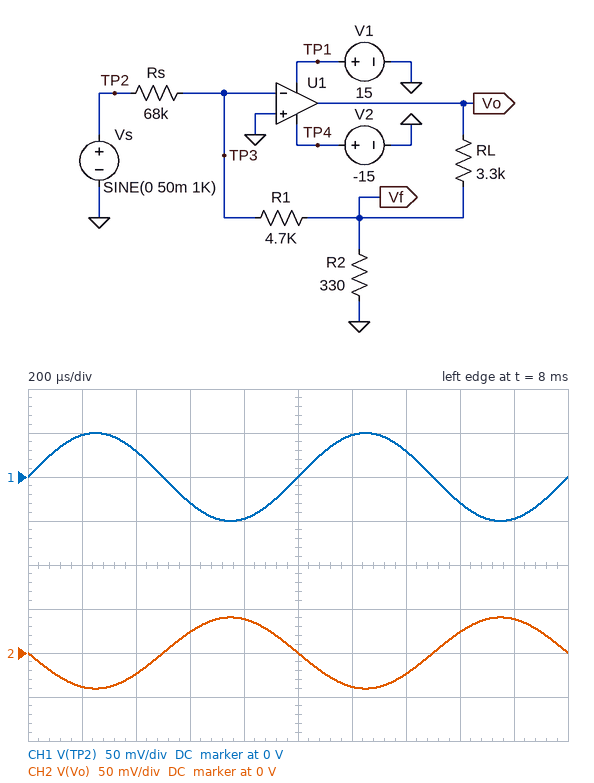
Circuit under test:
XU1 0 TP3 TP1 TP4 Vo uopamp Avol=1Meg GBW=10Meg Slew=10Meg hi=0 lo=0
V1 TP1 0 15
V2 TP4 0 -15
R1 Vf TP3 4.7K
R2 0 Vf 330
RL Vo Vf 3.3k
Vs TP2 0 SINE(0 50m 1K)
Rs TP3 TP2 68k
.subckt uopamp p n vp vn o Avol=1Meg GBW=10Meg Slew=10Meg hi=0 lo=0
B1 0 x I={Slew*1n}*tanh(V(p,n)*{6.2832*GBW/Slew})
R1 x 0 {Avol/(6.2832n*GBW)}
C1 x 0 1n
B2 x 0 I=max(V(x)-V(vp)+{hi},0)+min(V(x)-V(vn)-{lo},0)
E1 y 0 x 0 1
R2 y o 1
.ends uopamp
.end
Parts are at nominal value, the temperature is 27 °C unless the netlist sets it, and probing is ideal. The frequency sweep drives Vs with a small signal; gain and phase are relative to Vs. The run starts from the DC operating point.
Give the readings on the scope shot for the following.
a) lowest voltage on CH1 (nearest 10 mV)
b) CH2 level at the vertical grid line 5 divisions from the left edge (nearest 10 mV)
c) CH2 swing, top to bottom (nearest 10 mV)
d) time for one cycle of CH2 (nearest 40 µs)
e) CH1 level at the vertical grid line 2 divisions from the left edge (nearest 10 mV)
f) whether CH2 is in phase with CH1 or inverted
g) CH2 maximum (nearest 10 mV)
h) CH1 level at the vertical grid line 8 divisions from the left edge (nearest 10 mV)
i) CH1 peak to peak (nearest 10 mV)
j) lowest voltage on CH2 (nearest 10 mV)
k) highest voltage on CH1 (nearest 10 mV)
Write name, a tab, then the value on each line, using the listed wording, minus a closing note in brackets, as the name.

lowest voltage on CH1	-50 mV
CH2 level at the vertical grid line 5 divisions from the left edge	0 V
CH2 swing, top to bottom	80 mV
time for one cycle of CH2	1.00 ms
CH1 level at the vertical grid line 2 divisions from the left edge	30 mV
whether CH2 is in phase with CH1 or inverted	inverted
CH2 maximum	40 mV
CH1 level at the vertical grid line 8 divisions from the left edge	-30 mV
CH1 peak to peak	100 mV
lowest voltage on CH2	-40 mV
highest voltage on CH1	50 mV
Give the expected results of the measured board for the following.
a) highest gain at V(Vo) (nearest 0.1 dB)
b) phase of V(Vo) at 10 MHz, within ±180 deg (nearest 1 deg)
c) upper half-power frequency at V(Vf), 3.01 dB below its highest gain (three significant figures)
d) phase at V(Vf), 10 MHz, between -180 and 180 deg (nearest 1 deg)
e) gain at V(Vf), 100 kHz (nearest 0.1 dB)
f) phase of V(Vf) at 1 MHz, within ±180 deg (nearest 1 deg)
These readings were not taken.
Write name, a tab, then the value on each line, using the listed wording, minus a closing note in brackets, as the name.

highest gain at V(Vo)	-1.8 dB
phase of V(Vo) at 10 MHz, within ±180 deg	95 deg
upper half-power frequency at V(Vf), 3.01 dB below its highest gain	850 kHz
phase at V(Vf), 10 MHz, between -180 and 180 deg	60 deg
gain at V(Vf), 100 kHz	-23.3 dB
phase of V(Vf) at 1 MHz, within ±180 deg	126 deg
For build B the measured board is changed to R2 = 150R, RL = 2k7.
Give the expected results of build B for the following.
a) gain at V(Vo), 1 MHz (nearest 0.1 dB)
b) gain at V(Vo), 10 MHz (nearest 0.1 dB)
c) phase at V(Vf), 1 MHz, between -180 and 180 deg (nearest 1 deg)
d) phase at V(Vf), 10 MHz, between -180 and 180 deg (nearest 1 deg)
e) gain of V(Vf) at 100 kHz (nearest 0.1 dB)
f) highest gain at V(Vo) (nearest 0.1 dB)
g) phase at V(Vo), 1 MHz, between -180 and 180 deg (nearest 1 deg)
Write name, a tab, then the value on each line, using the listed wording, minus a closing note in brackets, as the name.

gain at V(Vo), 1 MHz	-4.5 dB
gain at V(Vo), 10 MHz	-23.6 dB
phase at V(Vf), 1 MHz, between -180 and 180 deg	113 deg
phase at V(Vf), 10 MHz, between -180 and 180 deg	63 deg
gain of V(Vf) at 100 kHz	-23.4 dB
highest gain at V(Vo)	2.6 dB
phase at V(Vo), 1 MHz, between -180 and 180 deg	116 deg
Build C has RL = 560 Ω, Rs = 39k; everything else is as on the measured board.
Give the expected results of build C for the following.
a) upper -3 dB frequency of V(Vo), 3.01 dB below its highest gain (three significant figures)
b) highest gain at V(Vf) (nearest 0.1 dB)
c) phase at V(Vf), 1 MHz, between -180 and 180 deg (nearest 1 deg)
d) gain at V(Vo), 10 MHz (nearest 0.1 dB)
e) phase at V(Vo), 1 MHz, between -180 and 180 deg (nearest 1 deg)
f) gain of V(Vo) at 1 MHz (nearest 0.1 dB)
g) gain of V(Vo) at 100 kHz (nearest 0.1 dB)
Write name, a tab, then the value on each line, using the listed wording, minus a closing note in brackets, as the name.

upper -3 dB frequency of V(Vo), 3.01 dB below its highest gain	3.29 MHz
highest gain at V(Vf)	-18.4 dB
phase at V(Vf), 1 MHz, between -180 and 180 deg	162 deg
gain at V(Vo), 10 MHz	-19.5 dB
phase at V(Vo), 1 MHz, between -180 and 180 deg	163 deg
gain of V(Vo) at 1 MHz	-9.8 dB
gain of V(Vo) at 100 kHz	-9.4 dB
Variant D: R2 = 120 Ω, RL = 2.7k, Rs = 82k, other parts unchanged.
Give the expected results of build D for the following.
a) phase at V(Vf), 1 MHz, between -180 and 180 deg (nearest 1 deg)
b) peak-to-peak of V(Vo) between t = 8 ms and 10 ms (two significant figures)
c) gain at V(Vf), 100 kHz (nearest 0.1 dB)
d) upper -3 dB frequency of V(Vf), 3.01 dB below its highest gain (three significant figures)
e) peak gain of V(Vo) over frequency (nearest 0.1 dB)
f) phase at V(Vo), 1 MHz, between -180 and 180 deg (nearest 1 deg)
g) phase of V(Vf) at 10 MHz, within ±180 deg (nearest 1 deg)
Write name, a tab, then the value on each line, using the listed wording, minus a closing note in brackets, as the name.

phase at V(Vf), 1 MHz, between -180 and 180 deg	109 deg
peak-to-peak of V(Vo) between t = 8 ms and 10 ms	140 mV
gain at V(Vf), 100 kHz	-25.1 dB
upper -3 dB frequency of V(Vf), 3.01 dB below its highest gain	402 kHz
peak gain of V(Vo) over frequency	2.8 dB
phase at V(Vo), 1 MHz, between -180 and 180 deg	112 deg
phase of V(Vf) at 10 MHz, within ±180 deg	62 deg
